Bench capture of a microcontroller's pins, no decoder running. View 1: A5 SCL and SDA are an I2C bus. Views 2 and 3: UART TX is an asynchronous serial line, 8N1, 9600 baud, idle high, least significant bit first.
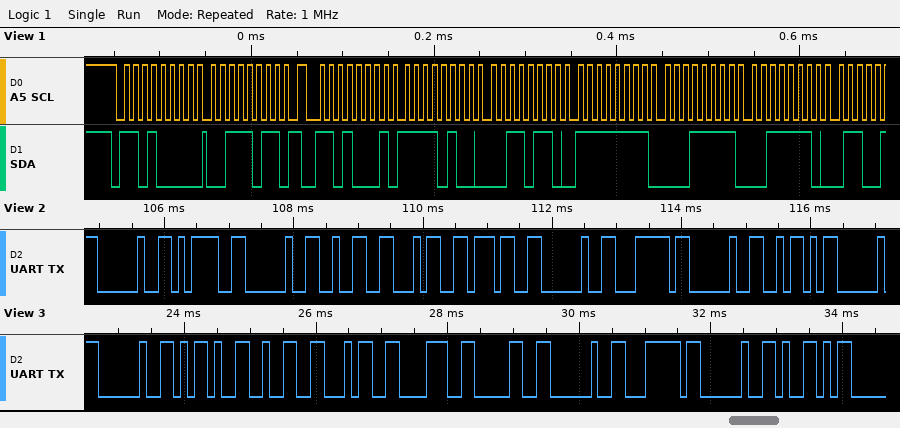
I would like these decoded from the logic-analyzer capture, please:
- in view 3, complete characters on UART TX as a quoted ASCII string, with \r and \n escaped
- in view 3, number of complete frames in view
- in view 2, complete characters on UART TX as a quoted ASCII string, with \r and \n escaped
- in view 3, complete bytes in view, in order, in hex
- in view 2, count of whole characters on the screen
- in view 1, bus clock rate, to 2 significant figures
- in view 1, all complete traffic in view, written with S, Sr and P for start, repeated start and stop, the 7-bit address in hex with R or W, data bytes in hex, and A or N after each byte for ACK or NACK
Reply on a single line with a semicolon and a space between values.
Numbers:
" -2480 | Y"; 10; " = 247 | Z"; 0x20 0x2D 0x32 0x34 0x38 0x30 0x20 0x7C 0x20 0x59; 10; 100 kHz; S 68W A 3B A Sr 68R A F4 A 36 A FF A 1F A 3E A
